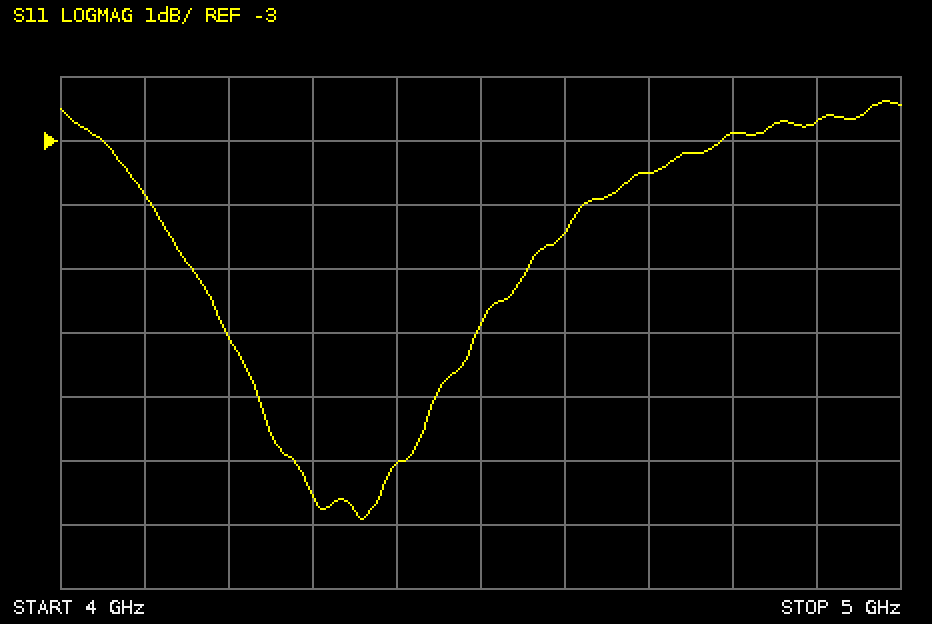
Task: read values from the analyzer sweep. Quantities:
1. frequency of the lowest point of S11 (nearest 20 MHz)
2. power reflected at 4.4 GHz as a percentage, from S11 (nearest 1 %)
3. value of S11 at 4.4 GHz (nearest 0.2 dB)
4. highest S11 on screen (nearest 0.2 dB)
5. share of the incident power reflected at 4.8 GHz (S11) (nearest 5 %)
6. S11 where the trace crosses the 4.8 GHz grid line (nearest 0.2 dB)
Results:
4.36 GHz
16 %
-8.0 dB
-2.4 dB
50 %
-2.8 dB
